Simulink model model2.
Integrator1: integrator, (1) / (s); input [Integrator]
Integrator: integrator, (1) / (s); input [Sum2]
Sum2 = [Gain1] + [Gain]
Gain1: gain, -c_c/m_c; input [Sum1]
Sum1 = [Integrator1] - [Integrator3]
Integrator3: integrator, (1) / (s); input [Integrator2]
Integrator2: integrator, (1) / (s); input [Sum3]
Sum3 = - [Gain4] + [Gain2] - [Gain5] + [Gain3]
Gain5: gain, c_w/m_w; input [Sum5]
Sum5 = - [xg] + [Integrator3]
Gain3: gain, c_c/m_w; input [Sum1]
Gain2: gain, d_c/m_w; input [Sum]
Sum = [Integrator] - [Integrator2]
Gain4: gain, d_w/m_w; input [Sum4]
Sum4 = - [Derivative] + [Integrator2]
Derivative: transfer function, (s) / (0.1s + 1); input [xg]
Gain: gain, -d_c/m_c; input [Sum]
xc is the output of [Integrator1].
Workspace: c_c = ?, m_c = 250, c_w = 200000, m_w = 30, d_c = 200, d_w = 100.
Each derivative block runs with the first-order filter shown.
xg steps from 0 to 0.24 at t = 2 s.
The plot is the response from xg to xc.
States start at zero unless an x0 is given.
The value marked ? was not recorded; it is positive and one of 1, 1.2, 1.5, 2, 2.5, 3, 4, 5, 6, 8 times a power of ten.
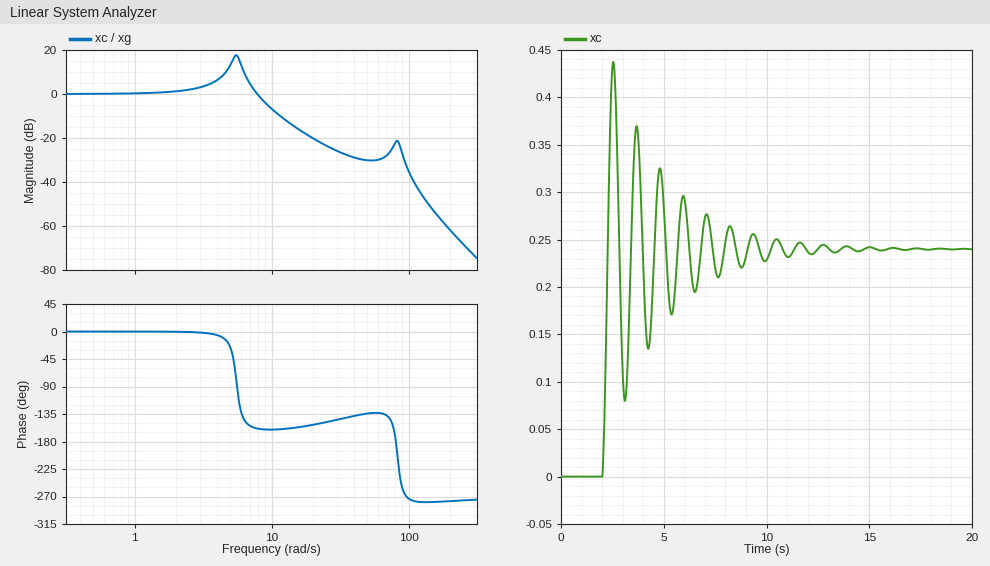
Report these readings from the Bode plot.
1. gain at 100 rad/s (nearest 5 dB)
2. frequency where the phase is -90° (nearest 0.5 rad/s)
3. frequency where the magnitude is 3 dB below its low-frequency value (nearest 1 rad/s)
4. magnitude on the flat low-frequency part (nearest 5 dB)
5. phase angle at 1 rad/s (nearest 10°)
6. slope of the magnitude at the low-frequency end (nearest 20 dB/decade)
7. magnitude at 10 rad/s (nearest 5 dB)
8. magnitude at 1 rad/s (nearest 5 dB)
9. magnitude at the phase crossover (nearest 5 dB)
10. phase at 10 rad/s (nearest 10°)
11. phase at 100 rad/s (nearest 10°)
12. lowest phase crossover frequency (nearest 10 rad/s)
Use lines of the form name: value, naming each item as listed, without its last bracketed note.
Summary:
gain at 100 rad/s: -35 dB
frequency where the phase is -90°: 5.5 rad/s
frequency where the magnitude is 3 dB below its low-frequency value: 9 rad/s
magnitude on the flat low-frequency part: 0 dB
phase angle at 1 rad/s: 0°
slope of the magnitude at the low-frequency end: 0 dB/decade
magnitude at 10 rad/s: -5 dB
magnitude at 1 rad/s: 0 dB
magnitude at the phase crossover: -20 dB
phase at 10 rad/s: -160°
phase at 100 rad/s: -270°
lowest phase crossover frequency: 80 rad/s
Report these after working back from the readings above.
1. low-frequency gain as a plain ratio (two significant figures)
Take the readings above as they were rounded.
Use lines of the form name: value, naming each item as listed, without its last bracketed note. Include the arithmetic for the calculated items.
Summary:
low-frequency gain as a plain ratio: 10^(0 / 20) = 1.0
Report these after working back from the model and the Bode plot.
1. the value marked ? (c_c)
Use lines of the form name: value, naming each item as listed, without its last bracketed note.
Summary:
the value marked ?: 8000
